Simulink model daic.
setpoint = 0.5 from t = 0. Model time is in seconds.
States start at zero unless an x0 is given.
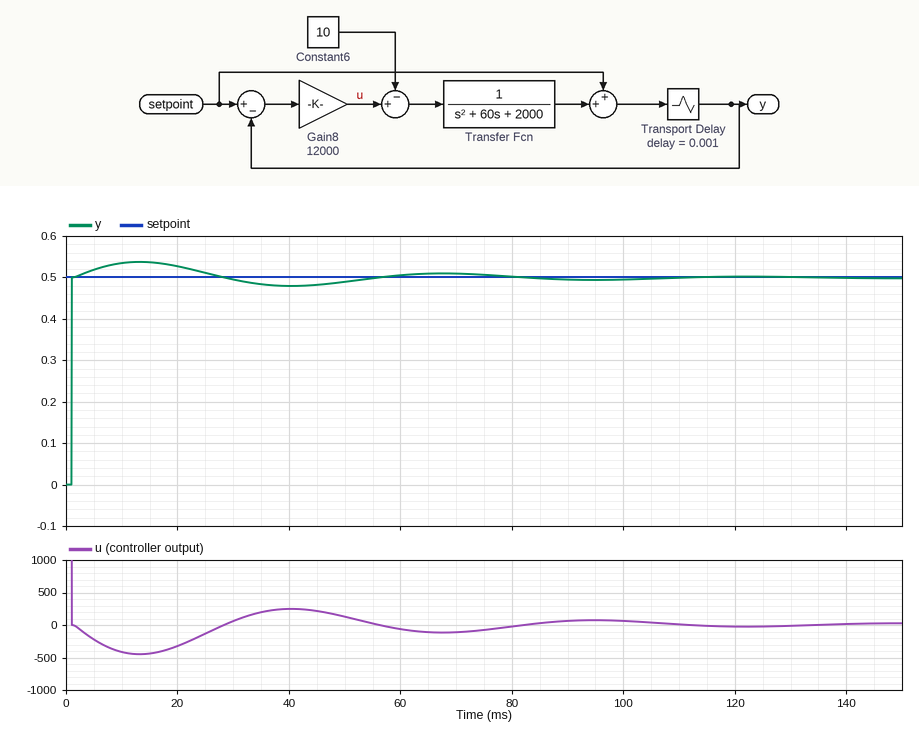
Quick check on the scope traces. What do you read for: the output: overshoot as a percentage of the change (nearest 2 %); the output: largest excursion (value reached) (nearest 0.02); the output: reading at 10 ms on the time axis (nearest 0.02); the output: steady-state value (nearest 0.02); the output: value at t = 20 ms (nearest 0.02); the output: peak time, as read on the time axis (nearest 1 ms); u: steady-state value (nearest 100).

8 %
0.54
0.54
0.50
0.52
13 ms
0
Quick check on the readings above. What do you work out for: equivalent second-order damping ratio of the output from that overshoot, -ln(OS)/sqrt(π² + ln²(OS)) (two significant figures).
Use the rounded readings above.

0.63
